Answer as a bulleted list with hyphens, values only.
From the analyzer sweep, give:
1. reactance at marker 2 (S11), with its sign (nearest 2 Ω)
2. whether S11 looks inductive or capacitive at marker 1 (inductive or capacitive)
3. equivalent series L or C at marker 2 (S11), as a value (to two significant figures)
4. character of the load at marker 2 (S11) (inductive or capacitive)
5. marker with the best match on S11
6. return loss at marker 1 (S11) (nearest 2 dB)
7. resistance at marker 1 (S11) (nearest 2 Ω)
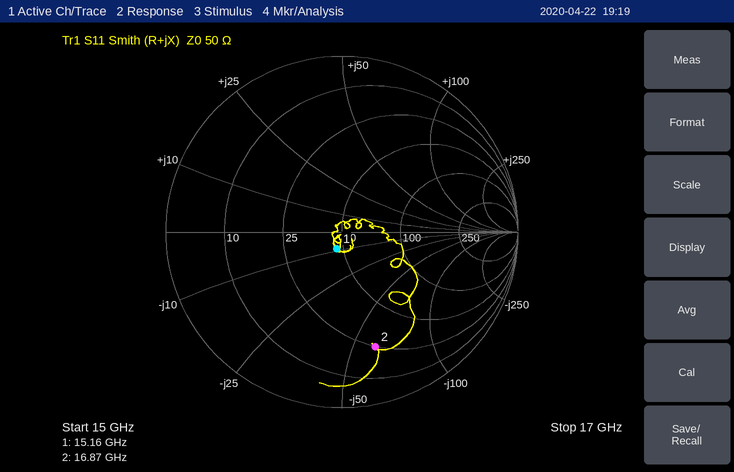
- -60 Ω
- capacitive
- 160 fF
- capacitive
- marker 1
- 20 dB
- 46 Ω
